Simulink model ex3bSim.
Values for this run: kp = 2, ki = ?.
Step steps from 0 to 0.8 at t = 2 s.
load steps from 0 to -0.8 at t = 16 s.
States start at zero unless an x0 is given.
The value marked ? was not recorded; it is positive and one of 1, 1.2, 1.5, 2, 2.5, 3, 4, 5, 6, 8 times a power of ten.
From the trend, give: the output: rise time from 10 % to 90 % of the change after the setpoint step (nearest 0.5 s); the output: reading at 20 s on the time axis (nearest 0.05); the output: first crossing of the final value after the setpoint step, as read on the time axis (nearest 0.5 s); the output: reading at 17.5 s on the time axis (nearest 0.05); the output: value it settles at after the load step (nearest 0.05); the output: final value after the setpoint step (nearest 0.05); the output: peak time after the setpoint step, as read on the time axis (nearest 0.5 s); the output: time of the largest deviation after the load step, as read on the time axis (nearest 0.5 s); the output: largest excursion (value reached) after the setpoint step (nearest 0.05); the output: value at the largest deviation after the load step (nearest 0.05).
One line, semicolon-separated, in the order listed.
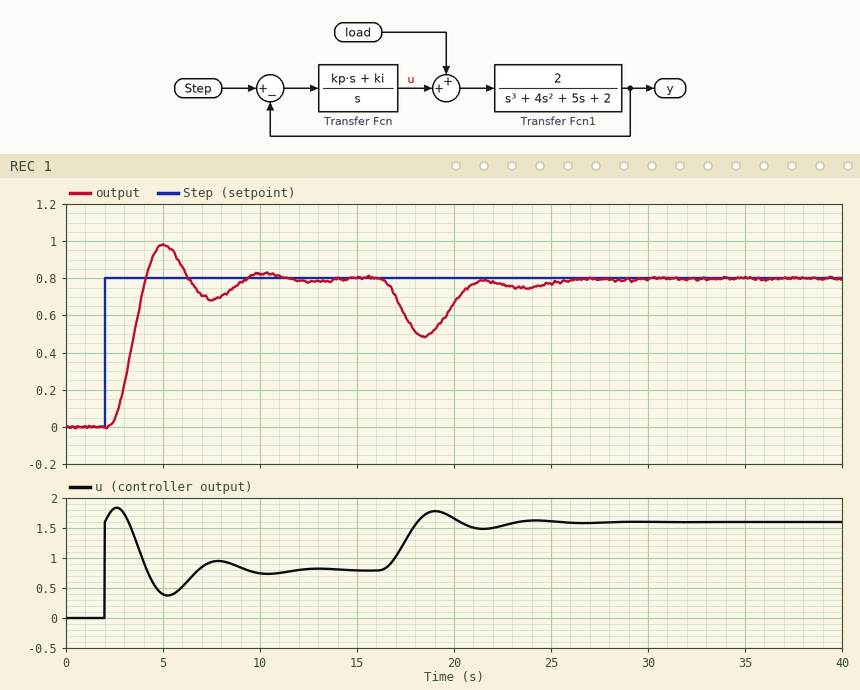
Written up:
1.5 s; 0.65; 4.0 s; 0.60; 0.80; 0.80; 5.0 s; 18.5 s; 1.00; 0.50
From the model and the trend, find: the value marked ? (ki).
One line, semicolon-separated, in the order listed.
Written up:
0.8
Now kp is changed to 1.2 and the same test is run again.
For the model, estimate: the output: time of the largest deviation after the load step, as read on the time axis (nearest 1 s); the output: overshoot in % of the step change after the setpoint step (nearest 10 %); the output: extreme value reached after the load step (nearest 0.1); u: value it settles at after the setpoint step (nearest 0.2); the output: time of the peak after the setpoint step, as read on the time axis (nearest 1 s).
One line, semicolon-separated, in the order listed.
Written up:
19 s; 20 %; 0.4; 0.8; 6 s
